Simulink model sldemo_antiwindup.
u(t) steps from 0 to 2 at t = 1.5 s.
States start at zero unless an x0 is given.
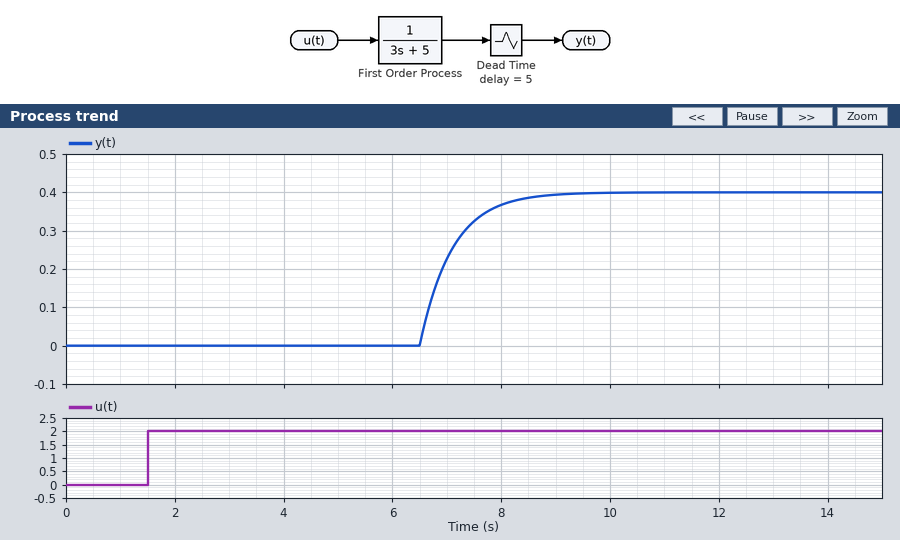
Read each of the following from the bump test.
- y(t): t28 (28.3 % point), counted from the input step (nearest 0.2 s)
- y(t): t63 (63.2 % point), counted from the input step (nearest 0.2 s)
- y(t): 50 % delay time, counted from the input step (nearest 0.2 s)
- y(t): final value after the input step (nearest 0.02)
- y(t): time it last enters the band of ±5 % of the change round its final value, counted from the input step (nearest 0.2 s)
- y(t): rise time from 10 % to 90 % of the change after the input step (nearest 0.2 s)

5.2 s
5.6 s
5.4 s
0.40
6.8 s
1.4 s
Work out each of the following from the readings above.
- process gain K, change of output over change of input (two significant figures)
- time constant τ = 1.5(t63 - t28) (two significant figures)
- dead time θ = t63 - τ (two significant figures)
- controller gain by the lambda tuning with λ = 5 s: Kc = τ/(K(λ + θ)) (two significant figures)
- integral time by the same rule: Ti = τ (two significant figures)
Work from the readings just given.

0.20
0.60 s
5.0 s
0.30
0.60 s
